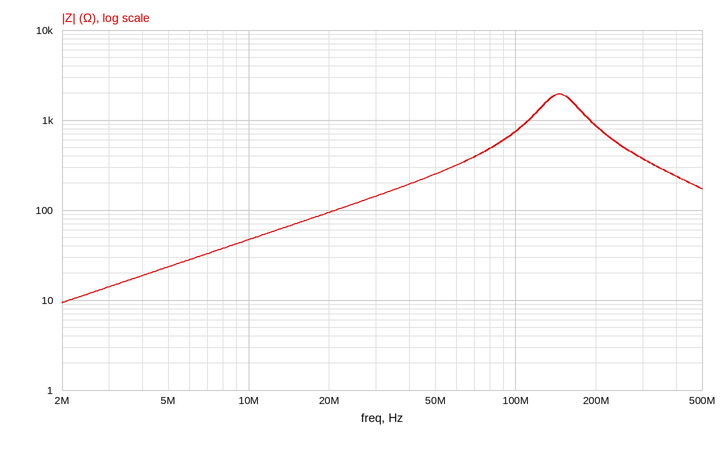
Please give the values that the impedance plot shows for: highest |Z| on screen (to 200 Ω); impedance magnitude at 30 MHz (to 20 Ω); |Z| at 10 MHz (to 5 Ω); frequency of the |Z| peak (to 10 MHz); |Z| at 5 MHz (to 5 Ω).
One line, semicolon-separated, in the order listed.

2.0 kΩ; 140 Ω; 45 Ω; 150 MHz; 25 Ω
